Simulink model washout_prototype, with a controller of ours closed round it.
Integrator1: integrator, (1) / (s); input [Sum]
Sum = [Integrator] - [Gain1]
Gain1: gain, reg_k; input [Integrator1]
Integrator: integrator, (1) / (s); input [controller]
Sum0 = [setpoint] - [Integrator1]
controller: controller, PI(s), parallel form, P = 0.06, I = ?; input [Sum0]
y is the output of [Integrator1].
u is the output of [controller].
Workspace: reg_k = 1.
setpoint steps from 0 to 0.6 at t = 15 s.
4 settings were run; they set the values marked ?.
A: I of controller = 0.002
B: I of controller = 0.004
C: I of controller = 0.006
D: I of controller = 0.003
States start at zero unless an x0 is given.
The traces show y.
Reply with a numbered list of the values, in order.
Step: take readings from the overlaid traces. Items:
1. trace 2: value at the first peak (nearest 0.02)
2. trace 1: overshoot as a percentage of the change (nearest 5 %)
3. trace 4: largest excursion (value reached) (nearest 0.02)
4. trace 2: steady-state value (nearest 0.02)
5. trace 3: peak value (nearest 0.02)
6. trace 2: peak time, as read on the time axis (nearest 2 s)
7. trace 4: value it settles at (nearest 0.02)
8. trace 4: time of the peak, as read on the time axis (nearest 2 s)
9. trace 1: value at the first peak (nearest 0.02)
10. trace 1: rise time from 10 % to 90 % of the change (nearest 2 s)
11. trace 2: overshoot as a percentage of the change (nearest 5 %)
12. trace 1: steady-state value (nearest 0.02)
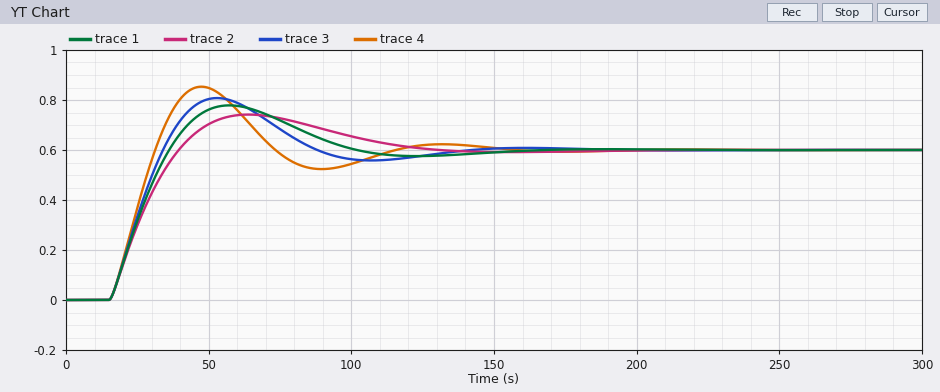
1. 0.74
2. 30 %
3. 0.86
4. 0.60
5. 0.80
6. 64 s
7. 0.60
8. 48 s
9. 0.78
10. 16 s
11. 25 %
12. 0.60
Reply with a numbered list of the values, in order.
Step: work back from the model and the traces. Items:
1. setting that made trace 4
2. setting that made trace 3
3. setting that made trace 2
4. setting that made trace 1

1. C
2. B
3. A
4. D
